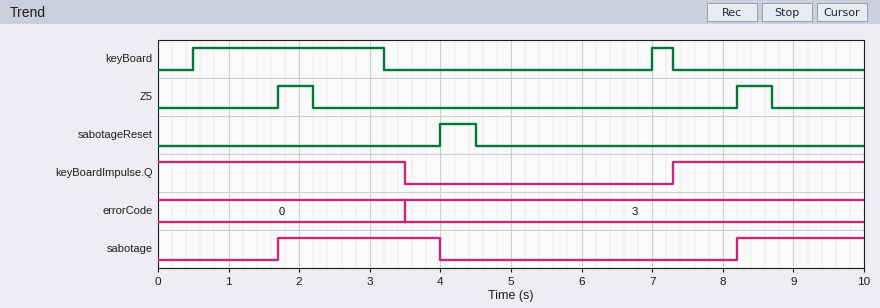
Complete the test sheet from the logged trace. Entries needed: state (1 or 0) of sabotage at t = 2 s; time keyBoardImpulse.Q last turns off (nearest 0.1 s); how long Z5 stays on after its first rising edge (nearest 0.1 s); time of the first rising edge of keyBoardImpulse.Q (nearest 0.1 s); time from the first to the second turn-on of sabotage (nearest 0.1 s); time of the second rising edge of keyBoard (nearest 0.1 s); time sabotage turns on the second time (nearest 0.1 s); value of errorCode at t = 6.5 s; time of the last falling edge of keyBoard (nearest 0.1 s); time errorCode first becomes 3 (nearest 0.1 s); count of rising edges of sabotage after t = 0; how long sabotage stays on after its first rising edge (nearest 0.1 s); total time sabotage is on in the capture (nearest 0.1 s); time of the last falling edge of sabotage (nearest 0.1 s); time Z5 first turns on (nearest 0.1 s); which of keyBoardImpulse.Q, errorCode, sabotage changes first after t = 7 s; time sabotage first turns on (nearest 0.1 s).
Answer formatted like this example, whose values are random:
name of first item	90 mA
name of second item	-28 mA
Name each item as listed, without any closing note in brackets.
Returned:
state (1 or 0) of sabotage at t = 2 s	1
time keyBoardImpulse.Q last turns off	3.5 s
how long Z5 stays on after its first rising edge	0.5 s
time of the first rising edge of keyBoardImpulse.Q	7.3 s
time from the first to the second turn-on of sabotage	6.5 s
time of the second rising edge of keyBoard	7.0 s
time sabotage turns on the second time	8.2 s
value of errorCode at t = 6.5 s	3
time of the last falling edge of keyBoard	7.3 s
time errorCode first becomes 3	3.5 s
count of rising edges of sabotage after t = 0	2
how long sabotage stays on after its first rising edge	2.3 s
total time sabotage is on in the capture	4.1 s
time of the last falling edge of sabotage	4.0 s
time Z5 first turns on	1.7 s
which of keyBoardImpulse.Q, errorCode, sabotage changes first after t = 7 s	keyBoardImpulse.Q
time sabotage first turns on	1.7 s
